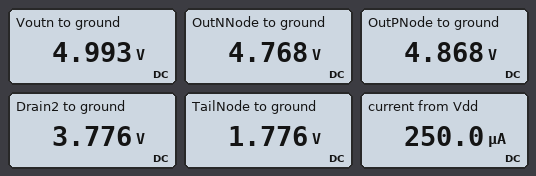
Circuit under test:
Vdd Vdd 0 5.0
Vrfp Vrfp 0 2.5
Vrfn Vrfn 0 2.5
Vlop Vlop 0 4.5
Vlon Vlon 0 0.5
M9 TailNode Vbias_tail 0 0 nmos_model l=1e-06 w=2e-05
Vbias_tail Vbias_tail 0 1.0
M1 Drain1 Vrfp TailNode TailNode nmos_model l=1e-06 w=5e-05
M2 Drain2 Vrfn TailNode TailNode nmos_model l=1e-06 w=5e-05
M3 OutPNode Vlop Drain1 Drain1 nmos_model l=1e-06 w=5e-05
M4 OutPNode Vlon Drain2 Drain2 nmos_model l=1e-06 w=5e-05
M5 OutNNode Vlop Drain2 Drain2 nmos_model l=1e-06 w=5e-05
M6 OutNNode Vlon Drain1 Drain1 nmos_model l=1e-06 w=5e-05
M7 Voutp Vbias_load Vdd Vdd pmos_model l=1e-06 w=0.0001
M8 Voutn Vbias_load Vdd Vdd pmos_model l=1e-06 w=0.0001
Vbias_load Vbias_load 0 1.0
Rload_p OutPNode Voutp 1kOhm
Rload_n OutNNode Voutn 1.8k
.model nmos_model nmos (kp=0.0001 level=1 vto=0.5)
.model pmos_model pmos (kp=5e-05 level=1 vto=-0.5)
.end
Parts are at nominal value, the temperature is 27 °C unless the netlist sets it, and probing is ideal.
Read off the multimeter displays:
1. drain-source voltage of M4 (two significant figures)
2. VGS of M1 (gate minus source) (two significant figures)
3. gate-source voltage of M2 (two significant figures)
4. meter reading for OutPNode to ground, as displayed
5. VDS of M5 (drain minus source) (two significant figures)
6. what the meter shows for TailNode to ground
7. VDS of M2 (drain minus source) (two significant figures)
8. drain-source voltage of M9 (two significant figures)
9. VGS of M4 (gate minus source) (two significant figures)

1.1 V
720 mV
720 mV
4.868 V
990 mV
1.776 V
2.0 V
1.8 V
-3.3 V
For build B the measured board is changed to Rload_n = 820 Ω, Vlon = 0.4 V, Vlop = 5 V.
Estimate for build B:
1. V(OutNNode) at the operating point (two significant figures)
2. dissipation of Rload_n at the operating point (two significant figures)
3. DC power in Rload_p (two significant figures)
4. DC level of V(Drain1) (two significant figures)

4.9 V
13 µW
16 µW
4.3 V
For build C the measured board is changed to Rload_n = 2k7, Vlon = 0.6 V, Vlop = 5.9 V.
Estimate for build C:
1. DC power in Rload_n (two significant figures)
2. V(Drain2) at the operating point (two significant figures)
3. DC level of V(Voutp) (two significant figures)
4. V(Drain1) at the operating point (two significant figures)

42 µW
4.6 V
5.0 V
4.8 V
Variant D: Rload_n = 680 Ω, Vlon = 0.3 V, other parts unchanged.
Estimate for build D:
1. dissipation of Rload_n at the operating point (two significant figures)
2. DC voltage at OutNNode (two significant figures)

11 µW
4.9 V
